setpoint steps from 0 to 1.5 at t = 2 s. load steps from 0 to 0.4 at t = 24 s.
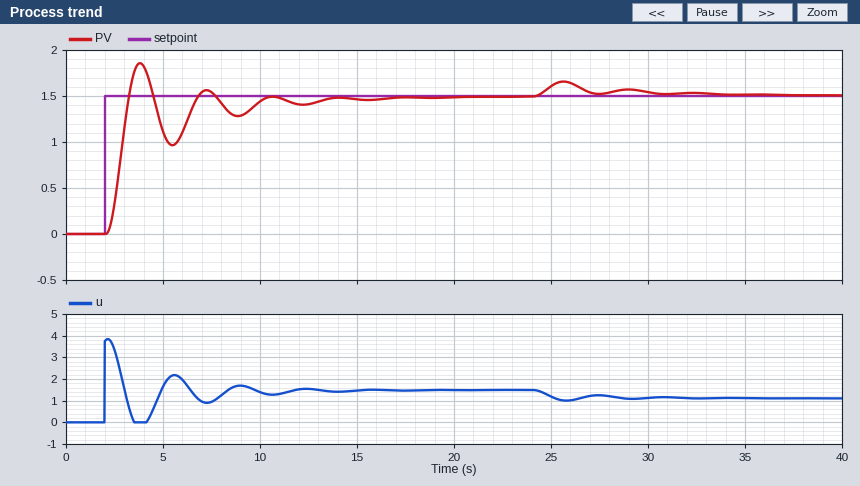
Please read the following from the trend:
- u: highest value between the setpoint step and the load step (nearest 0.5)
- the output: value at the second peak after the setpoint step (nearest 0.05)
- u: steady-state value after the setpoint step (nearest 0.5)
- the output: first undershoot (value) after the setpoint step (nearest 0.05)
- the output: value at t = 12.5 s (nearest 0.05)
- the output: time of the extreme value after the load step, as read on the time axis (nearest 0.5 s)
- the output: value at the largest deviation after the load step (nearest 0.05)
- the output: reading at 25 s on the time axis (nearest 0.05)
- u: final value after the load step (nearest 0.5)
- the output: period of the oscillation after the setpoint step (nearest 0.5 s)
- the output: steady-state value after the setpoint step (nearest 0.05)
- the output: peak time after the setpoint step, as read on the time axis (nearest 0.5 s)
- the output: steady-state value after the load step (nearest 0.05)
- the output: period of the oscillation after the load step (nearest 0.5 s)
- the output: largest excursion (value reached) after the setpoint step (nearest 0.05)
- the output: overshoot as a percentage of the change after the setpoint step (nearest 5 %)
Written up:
4.0
1.55
1.5
0.95
1.40
25.5 s
1.65
1.60
1.0
3.5 s
1.50
4.0 s
1.50
3.5 s
1.85
25 %
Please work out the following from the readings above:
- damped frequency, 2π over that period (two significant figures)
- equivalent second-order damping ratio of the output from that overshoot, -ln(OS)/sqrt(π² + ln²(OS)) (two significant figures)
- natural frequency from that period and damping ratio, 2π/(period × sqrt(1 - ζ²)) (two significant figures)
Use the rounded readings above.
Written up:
1.8 rad/s
0.40
2.0 rad/s
